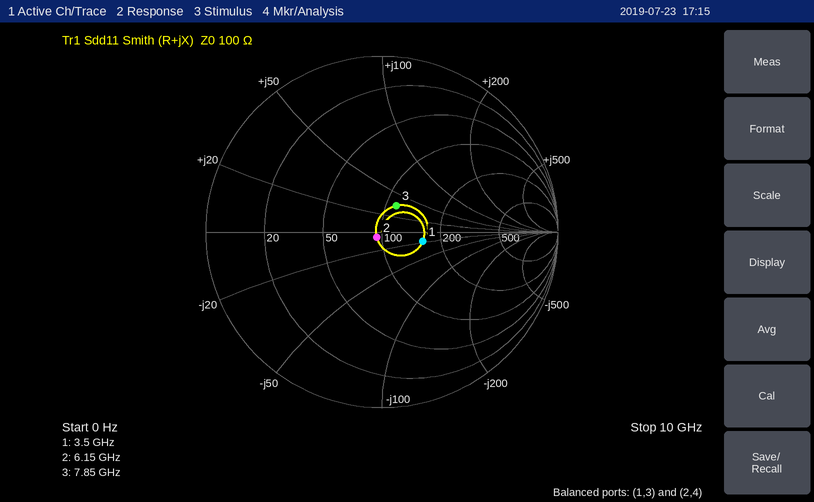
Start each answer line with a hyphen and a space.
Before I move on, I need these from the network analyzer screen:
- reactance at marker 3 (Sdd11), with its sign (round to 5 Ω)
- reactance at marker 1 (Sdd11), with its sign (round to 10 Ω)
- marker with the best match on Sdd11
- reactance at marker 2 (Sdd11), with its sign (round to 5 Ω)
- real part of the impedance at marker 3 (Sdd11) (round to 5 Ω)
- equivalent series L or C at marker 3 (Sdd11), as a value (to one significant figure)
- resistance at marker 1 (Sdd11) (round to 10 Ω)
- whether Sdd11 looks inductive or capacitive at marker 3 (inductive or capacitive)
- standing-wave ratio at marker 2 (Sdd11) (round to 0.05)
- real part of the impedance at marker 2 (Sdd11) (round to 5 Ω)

- +35 Ω
- -20 Ω
- marker 2
- -5 Ω
- 110 Ω
- 700 pH
- 160 Ω
- inductive
- 1.10
- 95 Ω
